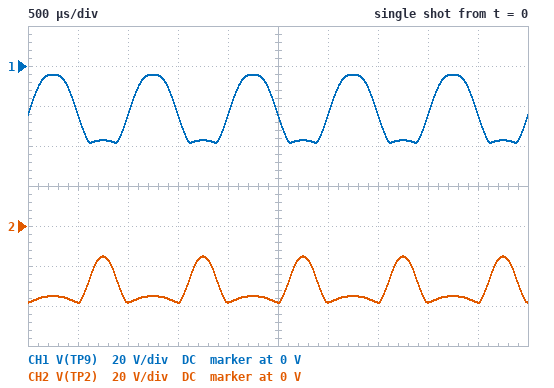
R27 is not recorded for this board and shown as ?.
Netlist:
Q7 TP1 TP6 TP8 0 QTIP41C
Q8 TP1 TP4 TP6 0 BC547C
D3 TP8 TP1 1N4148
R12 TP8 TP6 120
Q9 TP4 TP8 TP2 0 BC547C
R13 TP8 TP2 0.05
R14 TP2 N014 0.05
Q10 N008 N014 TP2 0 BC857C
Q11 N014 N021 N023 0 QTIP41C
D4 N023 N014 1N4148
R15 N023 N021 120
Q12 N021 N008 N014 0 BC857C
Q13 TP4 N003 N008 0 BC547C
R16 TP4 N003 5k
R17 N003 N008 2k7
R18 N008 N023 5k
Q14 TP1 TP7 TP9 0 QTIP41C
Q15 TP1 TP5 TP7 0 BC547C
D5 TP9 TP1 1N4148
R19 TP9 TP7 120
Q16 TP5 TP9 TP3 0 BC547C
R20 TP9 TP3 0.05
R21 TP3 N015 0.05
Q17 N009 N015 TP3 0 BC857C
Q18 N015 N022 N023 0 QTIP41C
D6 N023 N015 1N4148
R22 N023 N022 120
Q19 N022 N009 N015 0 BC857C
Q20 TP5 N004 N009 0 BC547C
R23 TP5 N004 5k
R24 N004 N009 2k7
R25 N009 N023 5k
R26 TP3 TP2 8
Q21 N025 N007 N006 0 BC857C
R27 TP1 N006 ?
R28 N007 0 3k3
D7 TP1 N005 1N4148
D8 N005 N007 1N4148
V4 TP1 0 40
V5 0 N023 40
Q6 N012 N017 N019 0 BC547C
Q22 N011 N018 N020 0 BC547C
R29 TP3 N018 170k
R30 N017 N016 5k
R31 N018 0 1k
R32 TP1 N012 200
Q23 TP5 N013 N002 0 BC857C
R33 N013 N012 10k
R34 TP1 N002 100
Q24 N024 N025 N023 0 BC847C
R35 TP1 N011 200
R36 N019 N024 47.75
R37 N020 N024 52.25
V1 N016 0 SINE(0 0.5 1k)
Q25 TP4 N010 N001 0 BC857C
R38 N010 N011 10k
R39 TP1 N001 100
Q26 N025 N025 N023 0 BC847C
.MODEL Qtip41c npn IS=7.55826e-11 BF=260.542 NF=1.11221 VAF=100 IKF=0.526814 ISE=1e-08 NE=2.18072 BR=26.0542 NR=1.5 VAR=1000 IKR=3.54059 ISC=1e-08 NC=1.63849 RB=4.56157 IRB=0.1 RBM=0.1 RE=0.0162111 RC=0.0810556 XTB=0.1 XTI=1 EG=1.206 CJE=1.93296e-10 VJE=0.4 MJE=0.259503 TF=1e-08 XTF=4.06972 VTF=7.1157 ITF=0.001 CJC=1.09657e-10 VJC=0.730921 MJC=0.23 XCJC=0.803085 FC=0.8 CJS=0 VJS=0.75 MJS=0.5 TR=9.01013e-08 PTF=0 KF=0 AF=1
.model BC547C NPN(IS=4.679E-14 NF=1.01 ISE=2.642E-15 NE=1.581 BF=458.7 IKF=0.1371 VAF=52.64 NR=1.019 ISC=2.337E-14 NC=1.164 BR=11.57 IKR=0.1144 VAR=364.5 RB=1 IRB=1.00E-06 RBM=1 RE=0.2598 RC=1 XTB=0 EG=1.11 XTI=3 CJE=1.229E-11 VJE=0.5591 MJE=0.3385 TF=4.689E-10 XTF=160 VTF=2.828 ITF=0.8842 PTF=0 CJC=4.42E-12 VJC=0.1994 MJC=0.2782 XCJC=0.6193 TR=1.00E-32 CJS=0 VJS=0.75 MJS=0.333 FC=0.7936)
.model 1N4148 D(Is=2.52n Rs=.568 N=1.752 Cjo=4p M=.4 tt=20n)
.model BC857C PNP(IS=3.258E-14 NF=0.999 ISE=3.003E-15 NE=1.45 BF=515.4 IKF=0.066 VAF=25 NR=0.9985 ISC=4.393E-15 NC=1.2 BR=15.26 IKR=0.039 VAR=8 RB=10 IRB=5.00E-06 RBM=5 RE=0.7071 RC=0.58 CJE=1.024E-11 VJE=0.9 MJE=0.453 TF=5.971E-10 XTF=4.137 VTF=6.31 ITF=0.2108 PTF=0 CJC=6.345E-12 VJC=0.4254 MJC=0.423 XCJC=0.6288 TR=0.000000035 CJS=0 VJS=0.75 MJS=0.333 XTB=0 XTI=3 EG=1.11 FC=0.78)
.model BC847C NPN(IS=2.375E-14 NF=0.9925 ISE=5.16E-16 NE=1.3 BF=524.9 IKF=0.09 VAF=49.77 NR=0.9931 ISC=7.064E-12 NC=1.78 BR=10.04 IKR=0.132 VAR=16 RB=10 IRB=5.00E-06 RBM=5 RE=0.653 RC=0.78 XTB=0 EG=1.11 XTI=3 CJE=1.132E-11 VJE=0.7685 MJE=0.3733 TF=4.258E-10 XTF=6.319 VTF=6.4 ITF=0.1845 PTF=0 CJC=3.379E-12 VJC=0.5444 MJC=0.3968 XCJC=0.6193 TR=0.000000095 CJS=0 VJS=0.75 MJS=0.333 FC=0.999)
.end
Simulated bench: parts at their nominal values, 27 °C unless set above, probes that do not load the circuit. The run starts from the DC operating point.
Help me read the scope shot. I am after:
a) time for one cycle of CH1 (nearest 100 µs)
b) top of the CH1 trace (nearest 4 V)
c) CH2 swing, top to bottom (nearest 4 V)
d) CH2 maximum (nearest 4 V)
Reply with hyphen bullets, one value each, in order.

- 1.0 ms
- -4 V
- 24 V
- -16 V
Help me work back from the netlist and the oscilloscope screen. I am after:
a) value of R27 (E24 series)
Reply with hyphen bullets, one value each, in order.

- 180 Ω
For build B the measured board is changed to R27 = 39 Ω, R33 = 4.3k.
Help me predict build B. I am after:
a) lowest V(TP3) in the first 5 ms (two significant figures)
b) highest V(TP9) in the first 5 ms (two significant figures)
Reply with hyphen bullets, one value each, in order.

- 11 V
- 37 V
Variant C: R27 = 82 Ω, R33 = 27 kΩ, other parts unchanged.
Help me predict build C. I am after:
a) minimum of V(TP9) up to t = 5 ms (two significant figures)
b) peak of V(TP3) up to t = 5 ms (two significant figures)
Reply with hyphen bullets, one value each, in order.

- -25 V
- 14 V
